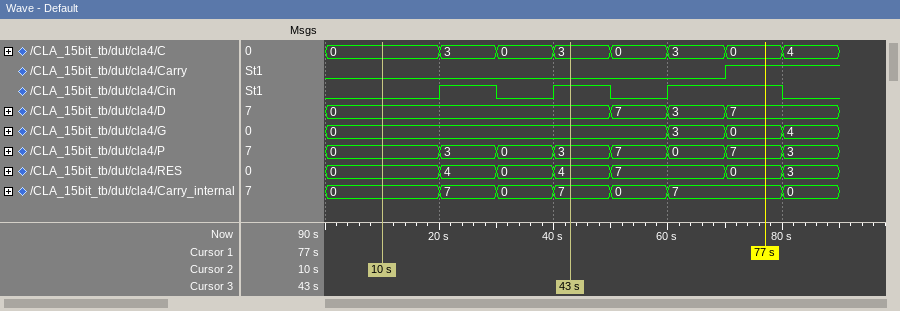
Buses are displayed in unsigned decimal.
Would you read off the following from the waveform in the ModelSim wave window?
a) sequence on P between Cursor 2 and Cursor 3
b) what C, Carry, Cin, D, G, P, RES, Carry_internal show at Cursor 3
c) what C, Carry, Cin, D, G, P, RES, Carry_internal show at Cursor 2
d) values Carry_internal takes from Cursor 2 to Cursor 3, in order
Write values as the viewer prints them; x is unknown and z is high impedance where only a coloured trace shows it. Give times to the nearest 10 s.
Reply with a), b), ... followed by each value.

a) 0, 3, 0, 3
b) C=3, Carry=0, Cin=1, D=0, G=0, P=3, RES=4, Carry_internal=7
c) C=0, Carry=0, Cin=0, D=0, G=0, P=0, RES=0, Carry_internal=0
d) 0, 7, 0, 7
